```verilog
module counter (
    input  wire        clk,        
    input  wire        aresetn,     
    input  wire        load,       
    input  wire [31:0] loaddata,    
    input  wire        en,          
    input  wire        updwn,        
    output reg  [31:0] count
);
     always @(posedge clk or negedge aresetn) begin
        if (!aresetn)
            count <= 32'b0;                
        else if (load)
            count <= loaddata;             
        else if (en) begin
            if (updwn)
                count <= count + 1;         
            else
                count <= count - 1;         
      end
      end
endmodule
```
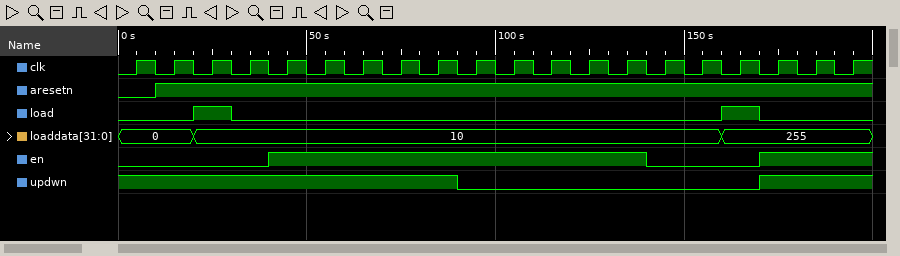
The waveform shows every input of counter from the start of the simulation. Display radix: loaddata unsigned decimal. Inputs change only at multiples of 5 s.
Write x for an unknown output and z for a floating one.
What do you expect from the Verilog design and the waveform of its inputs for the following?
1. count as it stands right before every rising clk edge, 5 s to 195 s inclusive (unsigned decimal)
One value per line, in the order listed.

0, 0, 0, 10, 10, 11, 12, 13, 14, 15, 14, 13, 12, 11, 10, 10, 10, 255, 256, 257
